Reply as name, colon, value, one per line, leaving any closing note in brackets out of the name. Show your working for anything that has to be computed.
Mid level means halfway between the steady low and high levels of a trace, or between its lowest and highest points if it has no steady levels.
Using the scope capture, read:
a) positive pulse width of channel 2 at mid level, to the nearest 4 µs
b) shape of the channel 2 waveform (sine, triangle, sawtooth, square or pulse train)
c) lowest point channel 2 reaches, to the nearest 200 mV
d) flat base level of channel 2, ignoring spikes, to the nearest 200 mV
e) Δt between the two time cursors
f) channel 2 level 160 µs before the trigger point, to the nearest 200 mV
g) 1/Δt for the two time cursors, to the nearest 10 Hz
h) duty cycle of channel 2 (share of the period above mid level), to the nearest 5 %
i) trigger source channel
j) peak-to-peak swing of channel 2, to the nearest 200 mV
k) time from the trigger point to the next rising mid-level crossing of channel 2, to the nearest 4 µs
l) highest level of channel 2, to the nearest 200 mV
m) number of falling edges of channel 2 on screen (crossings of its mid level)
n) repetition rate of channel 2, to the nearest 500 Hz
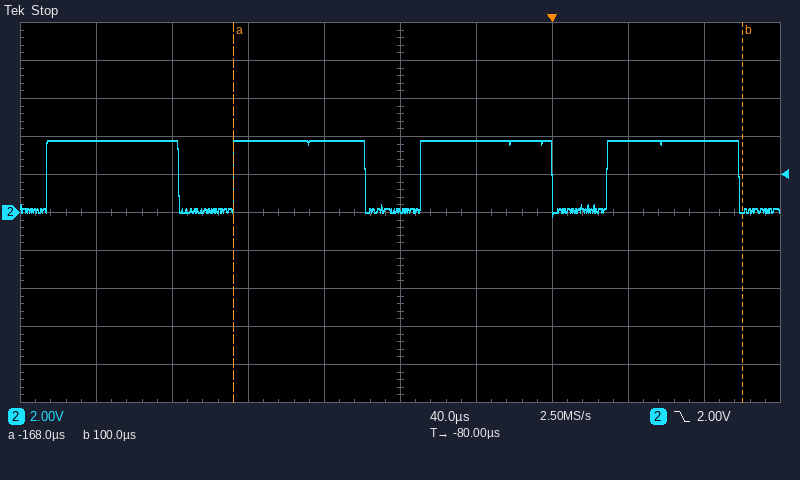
positive pulse width of channel 2 at mid level, to the nearest 4 µs: 68 µs
shape of the channel 2 waveform: pulse train
lowest point channel 2 reaches, to the nearest 200 mV: -200 mV
flat base level of channel 2, ignoring spikes, to the nearest 200 mV: 200 mV
Δt between the two time cursors: 100 µs − (-168 µs) = 268 µs
channel 2 level 160 µs before the trigger point, to the nearest 200 mV: 3.8 V
1/Δt for the two time cursors, to the nearest 10 Hz: 1 / 268 µs ≈ 3.73 kHz
duty cycle of channel 2 (share of the period above mid level), to the nearest 5 %: 70 %
trigger source channel: channel 2
peak-to-peak swing of channel 2, to the nearest 200 mV: 3.8 V − (-200 mV) = 4.0 V
time from the trigger point to the next rising mid-level crossing of channel 2, to the nearest 4 µs: 28 µs
highest level of channel 2, to the nearest 200 mV: 3.8 V
number of falling edges of channel 2 on screen: 4
repetition rate of channel 2, to the nearest 500 Hz: 10.0 kHz
